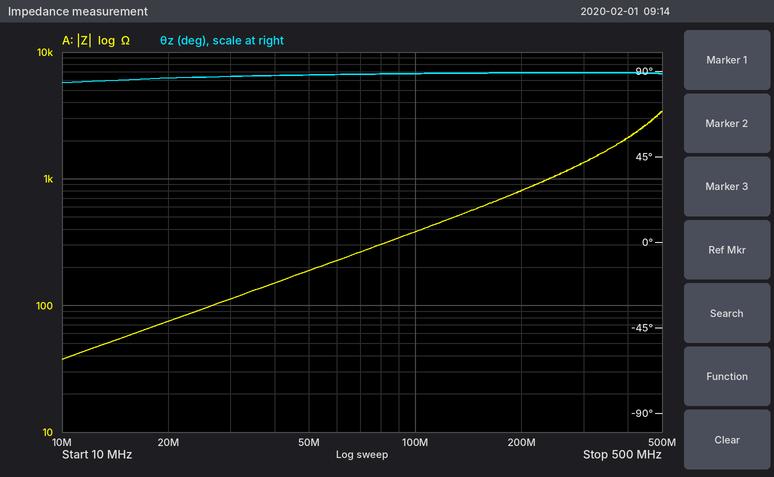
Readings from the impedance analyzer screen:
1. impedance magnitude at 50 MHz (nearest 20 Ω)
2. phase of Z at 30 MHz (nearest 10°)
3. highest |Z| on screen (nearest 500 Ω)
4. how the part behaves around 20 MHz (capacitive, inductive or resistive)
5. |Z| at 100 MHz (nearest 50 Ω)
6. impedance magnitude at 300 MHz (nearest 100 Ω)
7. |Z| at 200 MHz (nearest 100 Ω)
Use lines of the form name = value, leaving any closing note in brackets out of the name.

impedance magnitude at 50 MHz = 180 Ω
phase of Z at 30 MHz = 90°
highest |Z| on screen = 3.5 kΩ
how the part behaves around 20 MHz = inductive
|Z| at 100 MHz = 400 Ω
impedance magnitude at 300 MHz = 1.3 kΩ
|Z| at 200 MHz = 800 Ω
